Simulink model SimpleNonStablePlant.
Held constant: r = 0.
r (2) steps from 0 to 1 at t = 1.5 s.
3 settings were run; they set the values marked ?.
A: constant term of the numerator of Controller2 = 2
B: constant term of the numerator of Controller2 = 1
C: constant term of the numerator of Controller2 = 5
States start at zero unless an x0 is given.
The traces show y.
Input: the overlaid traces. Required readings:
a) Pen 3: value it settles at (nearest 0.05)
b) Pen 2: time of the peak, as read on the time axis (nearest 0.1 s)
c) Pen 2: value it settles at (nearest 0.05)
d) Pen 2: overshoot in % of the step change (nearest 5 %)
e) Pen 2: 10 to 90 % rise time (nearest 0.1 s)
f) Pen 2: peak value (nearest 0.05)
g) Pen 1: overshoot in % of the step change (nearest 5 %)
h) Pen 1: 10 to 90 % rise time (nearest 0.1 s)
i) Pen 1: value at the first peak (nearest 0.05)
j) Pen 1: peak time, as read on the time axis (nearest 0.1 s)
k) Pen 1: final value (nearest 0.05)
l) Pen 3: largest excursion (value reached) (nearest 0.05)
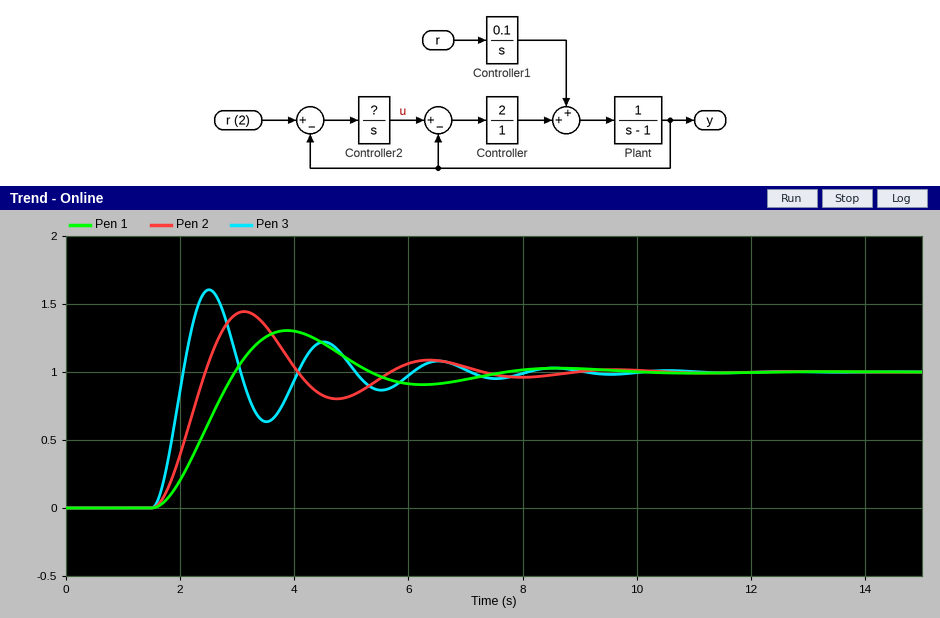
1.00
3.1 s
1.00
45 %
0.6 s
1.45
30 %
1.0 s
1.30
3.9 s
1.00
1.60
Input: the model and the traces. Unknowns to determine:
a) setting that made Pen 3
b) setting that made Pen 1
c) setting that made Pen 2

C
B
A
